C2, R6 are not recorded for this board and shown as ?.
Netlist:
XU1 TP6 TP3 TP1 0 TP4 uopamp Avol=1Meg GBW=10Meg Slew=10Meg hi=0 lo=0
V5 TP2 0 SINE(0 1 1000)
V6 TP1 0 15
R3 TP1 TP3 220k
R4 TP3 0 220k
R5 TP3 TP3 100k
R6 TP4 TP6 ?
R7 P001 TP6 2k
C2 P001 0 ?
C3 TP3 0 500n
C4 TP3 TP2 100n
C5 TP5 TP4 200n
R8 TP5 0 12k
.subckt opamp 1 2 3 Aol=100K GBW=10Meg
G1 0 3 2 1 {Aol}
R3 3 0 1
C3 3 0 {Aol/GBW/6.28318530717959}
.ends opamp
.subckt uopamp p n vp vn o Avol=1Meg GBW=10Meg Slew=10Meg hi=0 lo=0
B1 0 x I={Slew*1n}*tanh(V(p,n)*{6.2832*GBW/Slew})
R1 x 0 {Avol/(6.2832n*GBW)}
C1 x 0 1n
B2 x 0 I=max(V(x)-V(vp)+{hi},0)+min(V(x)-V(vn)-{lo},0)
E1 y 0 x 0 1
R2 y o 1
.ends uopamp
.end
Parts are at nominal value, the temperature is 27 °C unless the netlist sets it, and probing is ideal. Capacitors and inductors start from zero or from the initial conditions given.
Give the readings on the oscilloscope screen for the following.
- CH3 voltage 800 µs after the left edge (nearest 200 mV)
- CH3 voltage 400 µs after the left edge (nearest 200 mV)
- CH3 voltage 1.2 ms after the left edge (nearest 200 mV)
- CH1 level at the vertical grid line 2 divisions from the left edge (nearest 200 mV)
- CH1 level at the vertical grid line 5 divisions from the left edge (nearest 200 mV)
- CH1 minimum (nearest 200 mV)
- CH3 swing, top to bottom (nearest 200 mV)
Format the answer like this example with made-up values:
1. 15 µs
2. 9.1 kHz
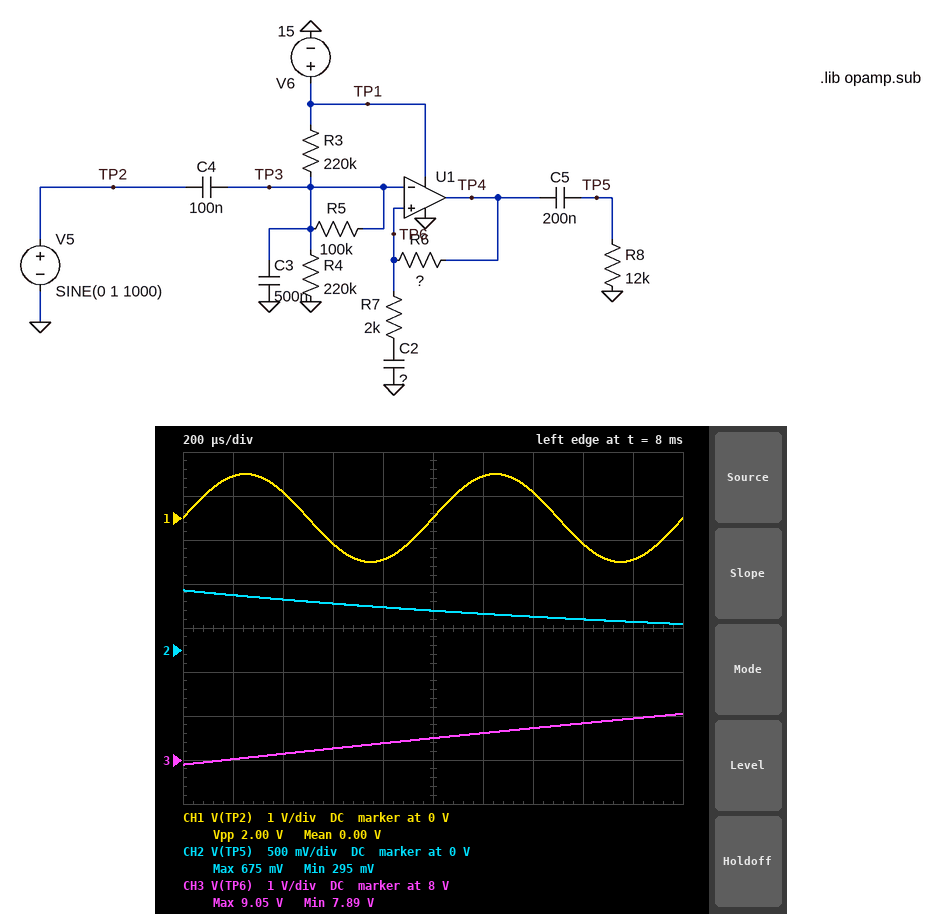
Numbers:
1. 8.4 V
2. 8.2 V
3. 8.6 V
4. 600 mV
5. 0 V
6. -1.0 V
7. 1.2 V
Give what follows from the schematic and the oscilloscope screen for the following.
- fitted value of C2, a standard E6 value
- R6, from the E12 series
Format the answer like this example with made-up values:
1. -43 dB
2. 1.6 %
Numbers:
1. 470 nF
2. 22 kΩ
